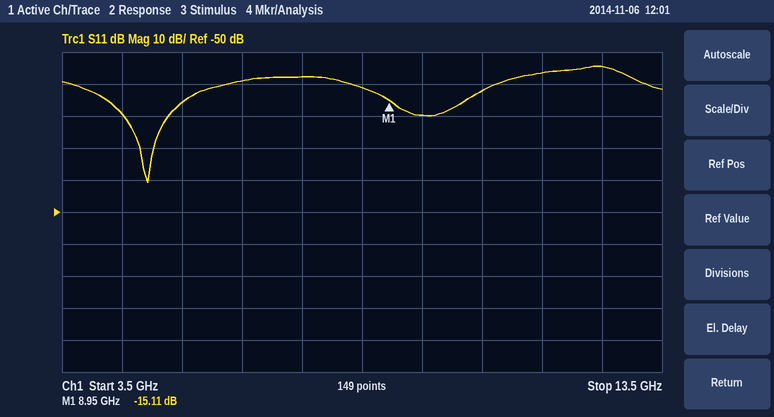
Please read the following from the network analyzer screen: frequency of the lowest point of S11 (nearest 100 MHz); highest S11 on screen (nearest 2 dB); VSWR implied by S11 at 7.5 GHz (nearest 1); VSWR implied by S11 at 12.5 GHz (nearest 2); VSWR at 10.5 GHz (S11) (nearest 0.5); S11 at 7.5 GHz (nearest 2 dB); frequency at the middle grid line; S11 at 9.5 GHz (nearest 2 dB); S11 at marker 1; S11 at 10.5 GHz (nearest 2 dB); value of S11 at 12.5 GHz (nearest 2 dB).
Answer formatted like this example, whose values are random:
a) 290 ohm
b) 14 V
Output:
a) 4.9 GHz
b) -4 dB
c) 2
d) 4
e) 1.5
f) -8 dB
g) 8.5 GHz
h) -20 dB
i) -15.11 dB
j) -12 dB
k) -4 dB
